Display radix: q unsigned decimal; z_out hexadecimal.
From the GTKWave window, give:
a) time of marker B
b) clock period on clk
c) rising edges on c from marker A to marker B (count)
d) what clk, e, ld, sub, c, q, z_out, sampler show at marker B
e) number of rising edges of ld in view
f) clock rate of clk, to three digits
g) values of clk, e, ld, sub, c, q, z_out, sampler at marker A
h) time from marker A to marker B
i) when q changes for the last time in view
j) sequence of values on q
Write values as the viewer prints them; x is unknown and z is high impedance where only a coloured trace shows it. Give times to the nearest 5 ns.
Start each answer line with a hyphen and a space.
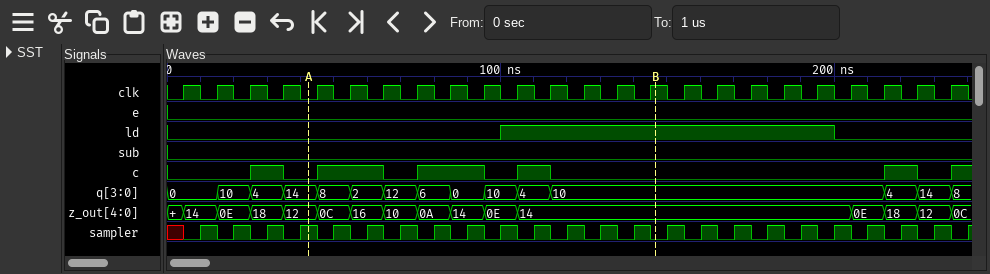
- 145 ns
- 10 ns
- 3
- clk=1, e=0, ld=1, sub=0, c=0, q=10, z_out=14, sampler=0
- 1
- 100 MHz
- clk=0, e=0, ld=0, sub=0, c=0, q=14, z_out=12, sampler=1
- 105 ns
- 235 ns
- 0, 10, 4, 14, 8, 2, 12, 6, 0, 10, 4, 10, 4, 14, 8
